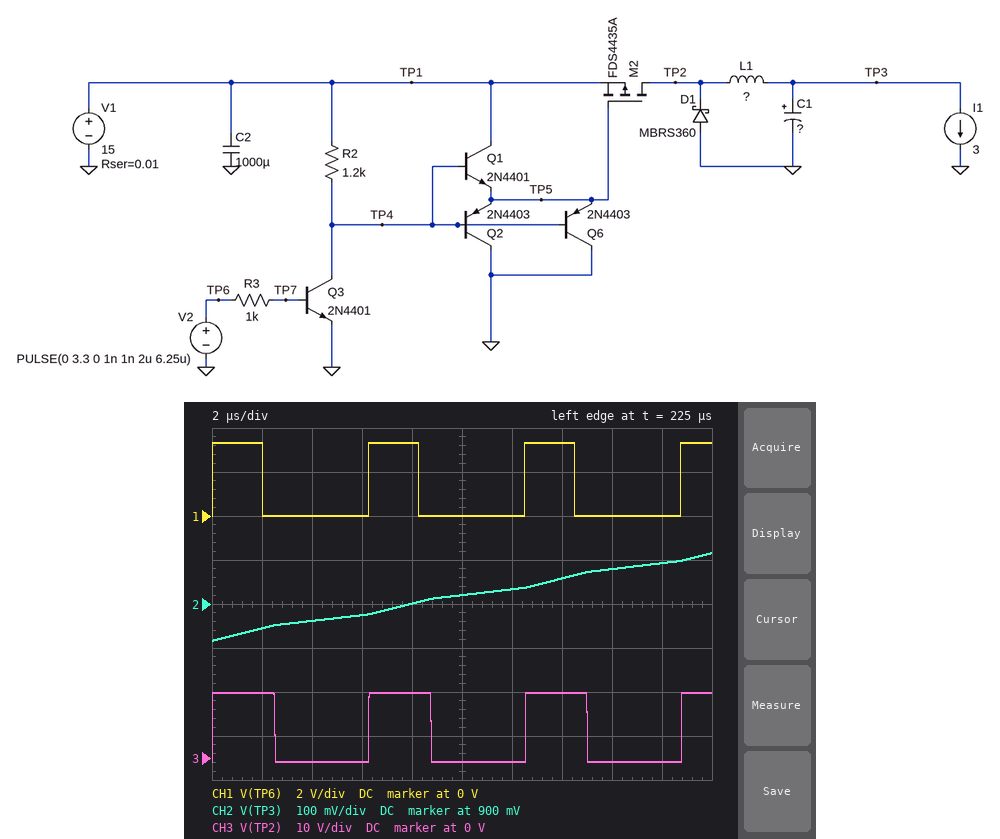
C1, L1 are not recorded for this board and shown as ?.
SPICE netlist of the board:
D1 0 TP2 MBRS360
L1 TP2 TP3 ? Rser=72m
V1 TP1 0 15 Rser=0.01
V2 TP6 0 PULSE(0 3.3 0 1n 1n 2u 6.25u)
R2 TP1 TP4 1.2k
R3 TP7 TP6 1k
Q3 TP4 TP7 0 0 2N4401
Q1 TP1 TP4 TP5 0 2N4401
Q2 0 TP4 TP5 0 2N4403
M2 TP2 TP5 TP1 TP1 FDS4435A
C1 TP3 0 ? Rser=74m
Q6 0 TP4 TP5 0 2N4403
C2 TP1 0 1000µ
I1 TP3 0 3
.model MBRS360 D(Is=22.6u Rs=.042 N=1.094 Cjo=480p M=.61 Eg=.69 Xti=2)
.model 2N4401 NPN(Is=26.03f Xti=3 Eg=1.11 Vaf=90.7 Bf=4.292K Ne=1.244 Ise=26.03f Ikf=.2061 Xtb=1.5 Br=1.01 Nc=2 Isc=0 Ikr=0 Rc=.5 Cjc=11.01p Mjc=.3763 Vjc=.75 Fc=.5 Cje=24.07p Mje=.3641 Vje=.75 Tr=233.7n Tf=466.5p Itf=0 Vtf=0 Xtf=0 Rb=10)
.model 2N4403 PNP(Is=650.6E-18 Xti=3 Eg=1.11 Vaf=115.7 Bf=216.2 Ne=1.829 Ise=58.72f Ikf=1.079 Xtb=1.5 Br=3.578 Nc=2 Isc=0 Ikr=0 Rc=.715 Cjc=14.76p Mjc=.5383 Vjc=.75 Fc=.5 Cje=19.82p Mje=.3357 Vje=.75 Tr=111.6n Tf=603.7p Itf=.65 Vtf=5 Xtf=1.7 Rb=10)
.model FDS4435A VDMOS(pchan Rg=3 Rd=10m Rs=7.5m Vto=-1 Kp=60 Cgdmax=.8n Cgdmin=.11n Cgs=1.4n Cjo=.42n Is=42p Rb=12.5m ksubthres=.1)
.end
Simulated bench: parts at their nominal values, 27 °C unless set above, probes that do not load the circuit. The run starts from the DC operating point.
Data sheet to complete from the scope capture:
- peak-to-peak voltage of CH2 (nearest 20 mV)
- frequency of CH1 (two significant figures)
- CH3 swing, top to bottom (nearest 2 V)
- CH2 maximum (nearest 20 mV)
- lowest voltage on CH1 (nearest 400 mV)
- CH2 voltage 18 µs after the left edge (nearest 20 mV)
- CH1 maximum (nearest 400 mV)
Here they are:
200 mV
160 kHz
16 V
1.02 V
0 V
1.00 V
3.2 V
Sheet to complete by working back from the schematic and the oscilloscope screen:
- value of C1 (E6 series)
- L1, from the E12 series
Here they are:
1 mF
150 µH
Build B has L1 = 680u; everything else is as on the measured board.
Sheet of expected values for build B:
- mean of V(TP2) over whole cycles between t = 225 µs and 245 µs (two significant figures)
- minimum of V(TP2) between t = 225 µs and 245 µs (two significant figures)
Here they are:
5.6 V
-560 mV
